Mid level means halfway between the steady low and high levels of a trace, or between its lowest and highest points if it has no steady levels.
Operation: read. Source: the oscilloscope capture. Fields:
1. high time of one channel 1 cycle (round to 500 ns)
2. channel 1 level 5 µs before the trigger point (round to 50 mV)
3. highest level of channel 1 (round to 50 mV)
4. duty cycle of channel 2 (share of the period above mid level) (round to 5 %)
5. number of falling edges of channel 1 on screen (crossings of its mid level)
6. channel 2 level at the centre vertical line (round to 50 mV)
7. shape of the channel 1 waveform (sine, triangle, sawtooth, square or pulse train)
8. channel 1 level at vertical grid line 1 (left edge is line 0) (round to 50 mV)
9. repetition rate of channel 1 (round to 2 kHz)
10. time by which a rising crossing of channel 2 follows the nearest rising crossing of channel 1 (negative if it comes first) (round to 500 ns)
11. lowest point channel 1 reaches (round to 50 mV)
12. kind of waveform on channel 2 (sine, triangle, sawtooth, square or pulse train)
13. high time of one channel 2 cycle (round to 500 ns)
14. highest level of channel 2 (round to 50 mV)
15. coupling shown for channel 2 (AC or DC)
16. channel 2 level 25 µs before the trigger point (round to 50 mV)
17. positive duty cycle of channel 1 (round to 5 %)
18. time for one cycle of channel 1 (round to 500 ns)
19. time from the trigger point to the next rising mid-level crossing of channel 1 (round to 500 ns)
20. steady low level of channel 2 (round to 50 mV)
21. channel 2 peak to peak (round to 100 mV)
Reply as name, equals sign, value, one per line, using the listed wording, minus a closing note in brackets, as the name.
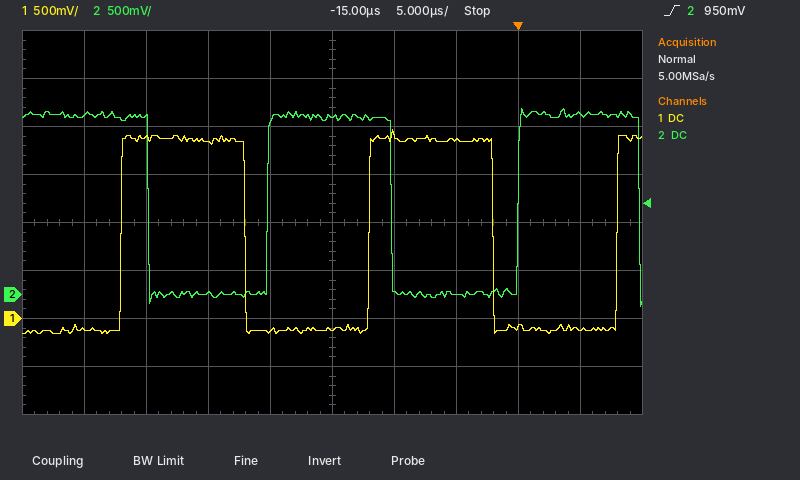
high time of one channel 1 cycle = 10.0 µs
channel 1 level 5 µs before the trigger point = 1.85 V
highest level of channel 1 = 1.95 V
duty cycle of channel 2 (share of the period above mid level) = 50 %
number of falling edges of channel 1 on screen = 2
channel 2 level at the centre vertical line = 1.85 V
shape of the channel 1 waveform = square
channel 1 level at vertical grid line 1 (left edge is line 0) = -100 mV
repetition rate of channel 1 = 50 kHz
time by which a rising crossing of channel 2 follows the nearest rising crossing of channel 1 (negative if it comes first) = -8.0 µs
lowest point channel 1 reaches = -150 mV
kind of waveform on channel 2 = square
high time of one channel 2 cycle = 10.0 µs
highest level of channel 2 = 1.95 V
coupling shown for channel 2 = DC
channel 2 level 25 µs before the trigger point = 0 mV
positive duty cycle of channel 1 = 50 %
time for one cycle of channel 1 = 20.0 µs
time from the trigger point to the next rising mid-level crossing of channel 1 = 8.0 µs
steady low level of channel 2 = 0 mV
channel 2 peak to peak = 2.10 V
